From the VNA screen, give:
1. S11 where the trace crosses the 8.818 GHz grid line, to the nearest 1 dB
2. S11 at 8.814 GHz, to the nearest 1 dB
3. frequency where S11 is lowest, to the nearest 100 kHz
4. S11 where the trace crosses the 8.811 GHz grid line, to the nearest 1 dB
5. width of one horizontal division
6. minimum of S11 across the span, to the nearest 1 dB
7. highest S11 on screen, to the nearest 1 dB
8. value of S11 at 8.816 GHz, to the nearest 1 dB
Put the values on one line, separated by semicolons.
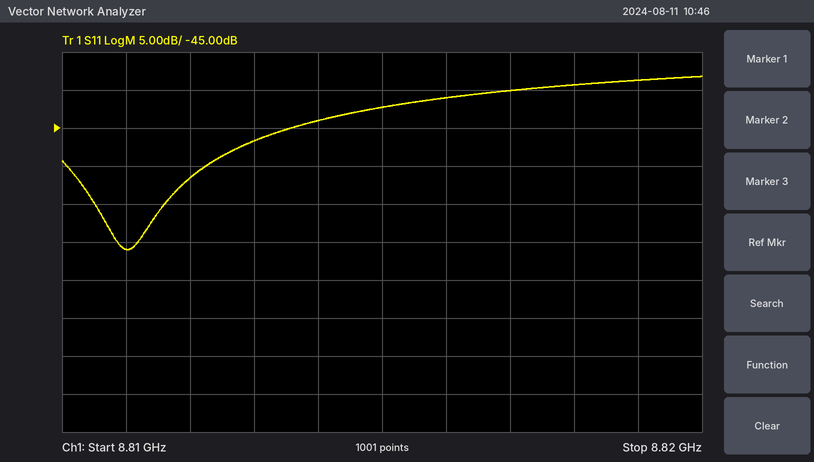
-39 dB; -44 dB; 8.8110 GHz; -61 dB; 1 MHz; -61 dB; -38 dB; -41 dB
